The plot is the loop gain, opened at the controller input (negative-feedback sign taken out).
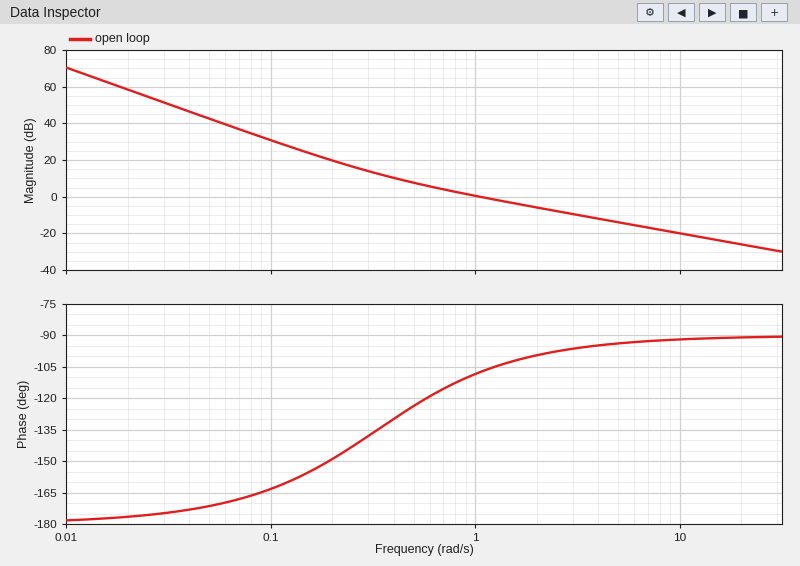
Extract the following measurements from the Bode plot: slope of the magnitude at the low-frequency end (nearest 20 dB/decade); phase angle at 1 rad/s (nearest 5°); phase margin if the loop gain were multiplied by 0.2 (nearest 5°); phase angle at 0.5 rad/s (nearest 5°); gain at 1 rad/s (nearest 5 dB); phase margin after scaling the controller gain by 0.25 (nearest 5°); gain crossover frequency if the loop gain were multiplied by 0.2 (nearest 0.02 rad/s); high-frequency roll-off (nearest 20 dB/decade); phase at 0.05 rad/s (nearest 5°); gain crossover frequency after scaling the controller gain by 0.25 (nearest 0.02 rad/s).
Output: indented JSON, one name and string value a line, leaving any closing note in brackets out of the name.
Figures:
{
  "slope of the magnitude at the low-frequency end": "-40 dB/decade",
  "phase angle at 1 rad/s": "-110°",
  "phase margin if the loop gain were multiplied by 0.2": "40°",
  "phase angle at 0.5 rad/s": "-125°",
  "gain at 1 rad/s": "0 dB",
  "phase margin after scaling the controller gain by 0.25": "45°",
  "gain crossover frequency if the loop gain were multiplied by 0.2": "0.30 rad/s",
  "high-frequency roll-off": "-20 dB/decade",
  "phase at 0.05 rad/s": "-170°",
  "gain crossover frequency after scaling the controller gain by 0.25": "0.34 rad/s"
}
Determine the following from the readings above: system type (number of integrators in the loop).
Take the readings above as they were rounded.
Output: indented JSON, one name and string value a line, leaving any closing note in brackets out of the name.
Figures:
{
  "system type": "2"
}
